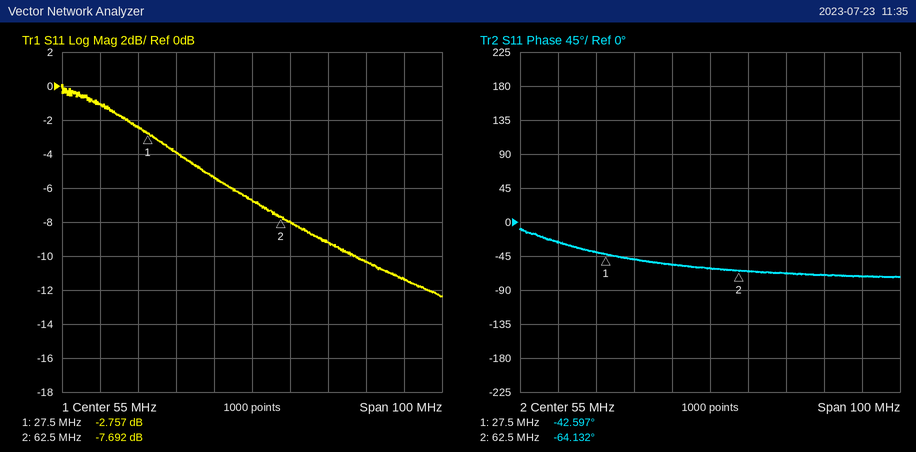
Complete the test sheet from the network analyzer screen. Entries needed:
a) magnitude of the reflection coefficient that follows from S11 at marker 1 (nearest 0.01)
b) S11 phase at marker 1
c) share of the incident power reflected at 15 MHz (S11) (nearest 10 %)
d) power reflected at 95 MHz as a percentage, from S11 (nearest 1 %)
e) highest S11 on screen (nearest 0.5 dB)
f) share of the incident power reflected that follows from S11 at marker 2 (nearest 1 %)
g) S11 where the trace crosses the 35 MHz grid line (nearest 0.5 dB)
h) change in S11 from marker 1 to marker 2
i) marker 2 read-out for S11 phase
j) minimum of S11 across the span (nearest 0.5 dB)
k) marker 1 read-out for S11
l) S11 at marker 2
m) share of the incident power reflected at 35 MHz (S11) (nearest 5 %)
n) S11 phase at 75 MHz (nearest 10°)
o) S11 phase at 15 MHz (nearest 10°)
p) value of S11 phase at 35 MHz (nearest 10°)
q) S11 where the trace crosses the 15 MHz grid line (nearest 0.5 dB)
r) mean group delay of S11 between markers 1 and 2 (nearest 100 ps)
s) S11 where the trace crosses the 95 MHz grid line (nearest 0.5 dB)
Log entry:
0.73
-42.597°
80 %
7 %
0.0 dB
17 %
-4.0 dB
-4.935 dB
-64.132°
-12.5 dB
-2.757 dB
-7.692 dB
40 %
-70°
-30°
-50°
-1.0 dB
1.7 ns
-11.5 dB
